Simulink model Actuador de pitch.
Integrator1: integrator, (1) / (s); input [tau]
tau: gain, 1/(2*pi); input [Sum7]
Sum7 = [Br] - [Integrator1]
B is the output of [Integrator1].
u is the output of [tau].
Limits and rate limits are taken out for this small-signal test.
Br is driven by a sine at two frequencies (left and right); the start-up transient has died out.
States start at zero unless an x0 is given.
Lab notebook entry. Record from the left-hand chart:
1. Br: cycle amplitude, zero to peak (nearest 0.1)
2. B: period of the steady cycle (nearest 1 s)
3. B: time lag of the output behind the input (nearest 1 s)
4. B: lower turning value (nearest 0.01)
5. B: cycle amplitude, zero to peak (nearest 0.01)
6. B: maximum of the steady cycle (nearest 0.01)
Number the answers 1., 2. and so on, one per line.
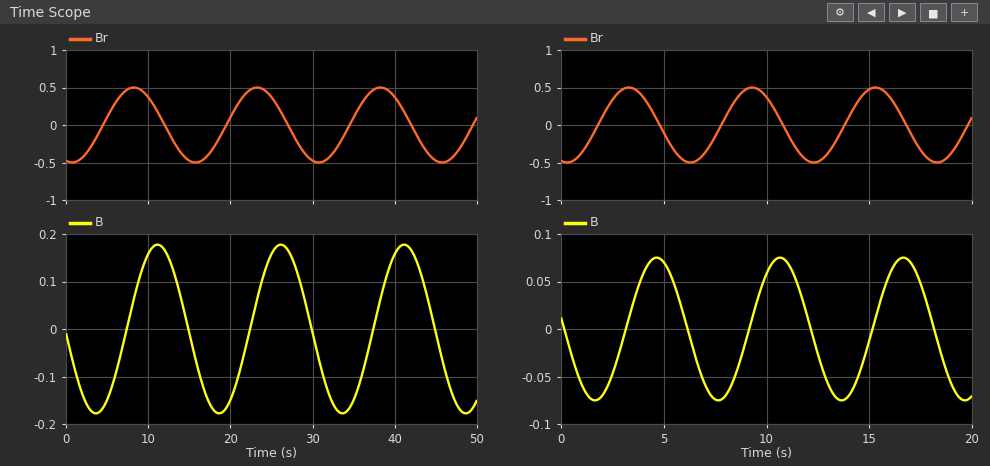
1. 0.5
2. 15 s
3. 3 s
4. -0.18
5. 0.18
6. 0.18
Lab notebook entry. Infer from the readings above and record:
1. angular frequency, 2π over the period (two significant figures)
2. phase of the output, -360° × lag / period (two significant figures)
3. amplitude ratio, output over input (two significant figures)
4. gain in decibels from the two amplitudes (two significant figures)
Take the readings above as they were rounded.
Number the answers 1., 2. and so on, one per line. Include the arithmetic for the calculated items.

1. 2π / 15 = 0.42 rad/s
2. -360 × 3 / 15 = -72°
3. 0.18 / 0.5 = 0.36
4. 20 log10(0.18 / 0.5) = -8.9 dB
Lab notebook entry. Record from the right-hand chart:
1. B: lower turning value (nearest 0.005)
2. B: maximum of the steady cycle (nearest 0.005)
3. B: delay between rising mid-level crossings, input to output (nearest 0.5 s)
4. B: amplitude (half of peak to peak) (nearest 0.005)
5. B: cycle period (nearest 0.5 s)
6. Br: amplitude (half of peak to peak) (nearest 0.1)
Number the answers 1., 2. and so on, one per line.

1. -0.075
2. 0.075
3. 1.5 s
4. 0.075
5. 6.0 s
6. 0.5
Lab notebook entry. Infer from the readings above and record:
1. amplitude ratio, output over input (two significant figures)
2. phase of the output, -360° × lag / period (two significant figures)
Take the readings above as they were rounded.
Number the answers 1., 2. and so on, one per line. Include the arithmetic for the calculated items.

1. 0.075 / 0.5 = 0.15
2. -360 × 1.5 / 6 = -90°
